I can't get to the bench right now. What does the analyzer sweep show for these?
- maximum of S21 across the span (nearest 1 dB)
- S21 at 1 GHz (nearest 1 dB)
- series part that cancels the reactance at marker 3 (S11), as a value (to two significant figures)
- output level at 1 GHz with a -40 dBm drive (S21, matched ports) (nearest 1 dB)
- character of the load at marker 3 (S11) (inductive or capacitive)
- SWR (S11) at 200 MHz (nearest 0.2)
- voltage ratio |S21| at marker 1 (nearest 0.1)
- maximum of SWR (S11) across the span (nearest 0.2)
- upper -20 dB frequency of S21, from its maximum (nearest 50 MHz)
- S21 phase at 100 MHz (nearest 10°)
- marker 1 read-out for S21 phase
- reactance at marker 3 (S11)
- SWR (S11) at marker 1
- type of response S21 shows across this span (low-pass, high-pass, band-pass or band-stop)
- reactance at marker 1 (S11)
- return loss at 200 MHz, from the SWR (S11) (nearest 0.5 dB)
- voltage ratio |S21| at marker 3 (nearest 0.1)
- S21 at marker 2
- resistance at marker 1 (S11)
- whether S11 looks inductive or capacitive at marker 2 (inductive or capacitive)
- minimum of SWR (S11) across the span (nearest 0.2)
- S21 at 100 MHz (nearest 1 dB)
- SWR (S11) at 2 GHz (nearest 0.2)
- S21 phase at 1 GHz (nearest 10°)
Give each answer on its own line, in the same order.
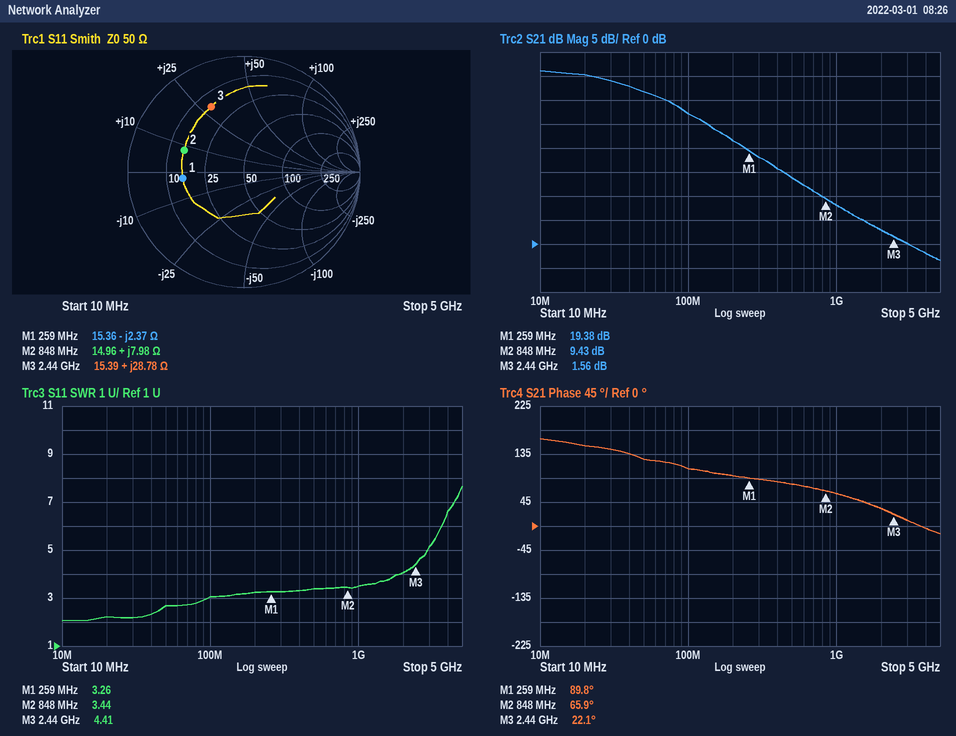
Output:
36 dB
8 dB
2.3 pF
-32 dBm
inductive
3.2
9.3
7.6
400 MHz
110°
89.8°
+28.78 Ω
3.26
low-pass
-2.37 Ω
5.5 dB
1.2
9.43 dB
15.36 Ω
inductive
2.0
27 dB
4.0
60°
